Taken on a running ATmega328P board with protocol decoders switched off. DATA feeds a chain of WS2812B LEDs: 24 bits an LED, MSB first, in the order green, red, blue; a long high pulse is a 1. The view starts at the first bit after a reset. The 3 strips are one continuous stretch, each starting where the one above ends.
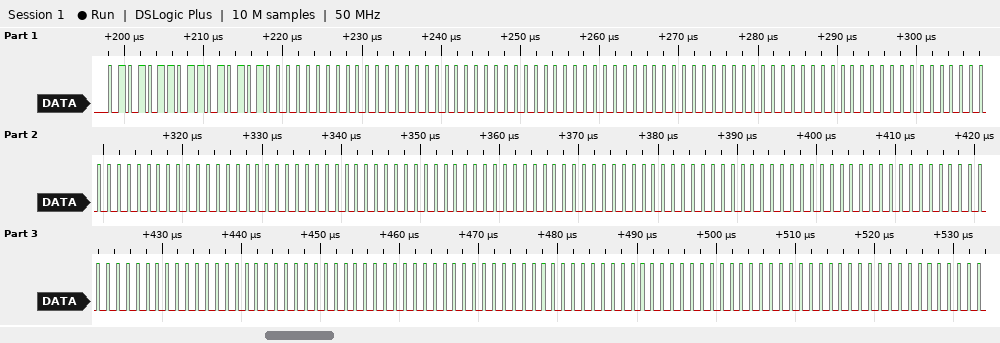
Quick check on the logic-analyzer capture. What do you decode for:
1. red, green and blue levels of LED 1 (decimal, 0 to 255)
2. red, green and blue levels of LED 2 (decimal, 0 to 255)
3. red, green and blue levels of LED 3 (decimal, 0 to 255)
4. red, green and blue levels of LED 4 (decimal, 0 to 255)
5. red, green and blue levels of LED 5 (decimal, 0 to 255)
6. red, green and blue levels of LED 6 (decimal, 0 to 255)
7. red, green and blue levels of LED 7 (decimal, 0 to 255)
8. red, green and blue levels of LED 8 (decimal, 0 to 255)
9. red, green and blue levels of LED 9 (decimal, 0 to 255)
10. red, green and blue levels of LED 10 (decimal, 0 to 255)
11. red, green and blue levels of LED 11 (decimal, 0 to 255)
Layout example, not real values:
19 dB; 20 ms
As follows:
213, 86, 0; 0, 0, 0; 0, 0, 0; 0, 0, 0; 0, 0, 0; 0, 0, 0; 0, 0, 0; 0, 0, 0; 0, 0, 0; 0, 0, 0; 0, 0, 0
